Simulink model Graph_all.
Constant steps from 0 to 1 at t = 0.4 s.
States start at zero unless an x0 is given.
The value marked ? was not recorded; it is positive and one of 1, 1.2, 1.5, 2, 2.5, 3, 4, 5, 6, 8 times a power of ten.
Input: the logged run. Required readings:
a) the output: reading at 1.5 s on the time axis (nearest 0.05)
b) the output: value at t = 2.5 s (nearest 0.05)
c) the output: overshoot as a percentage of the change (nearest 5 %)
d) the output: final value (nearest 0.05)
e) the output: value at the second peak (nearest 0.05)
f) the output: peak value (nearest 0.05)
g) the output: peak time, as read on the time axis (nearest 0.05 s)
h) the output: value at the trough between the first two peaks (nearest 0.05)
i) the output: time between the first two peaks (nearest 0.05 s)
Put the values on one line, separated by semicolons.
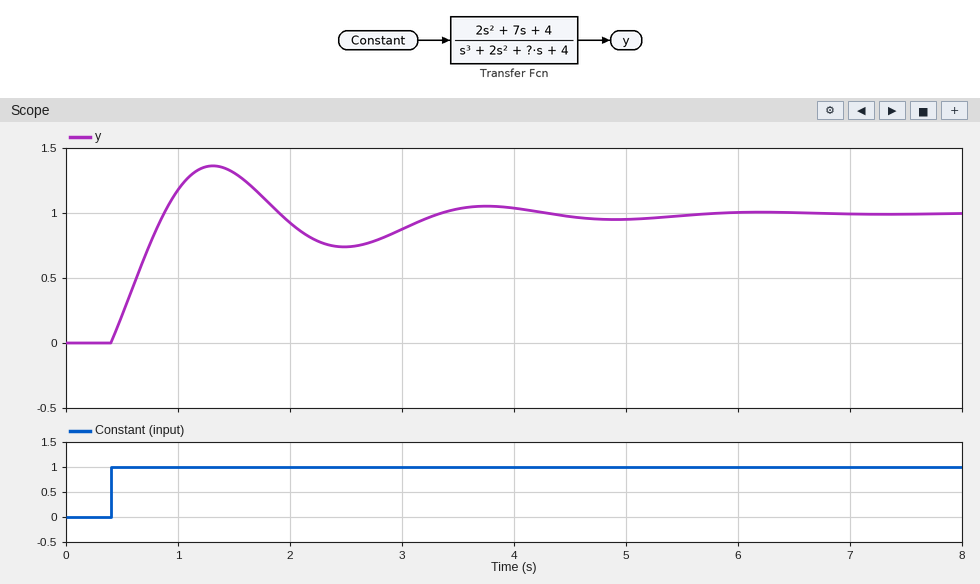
1.30; 0.75; 35 %; 1.00; 1.05; 1.35; 1.30 s; 0.75; 2.45 s
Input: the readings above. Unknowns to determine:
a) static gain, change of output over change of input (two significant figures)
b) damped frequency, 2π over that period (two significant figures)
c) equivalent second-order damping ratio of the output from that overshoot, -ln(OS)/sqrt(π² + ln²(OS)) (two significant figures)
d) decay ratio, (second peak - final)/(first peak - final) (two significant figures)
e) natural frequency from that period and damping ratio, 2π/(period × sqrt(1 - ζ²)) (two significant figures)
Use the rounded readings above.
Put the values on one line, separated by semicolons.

1.0; 2.6 rad/s; 0.32; 0.14; 2.7 rad/s
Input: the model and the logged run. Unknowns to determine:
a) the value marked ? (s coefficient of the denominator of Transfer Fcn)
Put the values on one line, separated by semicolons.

8
